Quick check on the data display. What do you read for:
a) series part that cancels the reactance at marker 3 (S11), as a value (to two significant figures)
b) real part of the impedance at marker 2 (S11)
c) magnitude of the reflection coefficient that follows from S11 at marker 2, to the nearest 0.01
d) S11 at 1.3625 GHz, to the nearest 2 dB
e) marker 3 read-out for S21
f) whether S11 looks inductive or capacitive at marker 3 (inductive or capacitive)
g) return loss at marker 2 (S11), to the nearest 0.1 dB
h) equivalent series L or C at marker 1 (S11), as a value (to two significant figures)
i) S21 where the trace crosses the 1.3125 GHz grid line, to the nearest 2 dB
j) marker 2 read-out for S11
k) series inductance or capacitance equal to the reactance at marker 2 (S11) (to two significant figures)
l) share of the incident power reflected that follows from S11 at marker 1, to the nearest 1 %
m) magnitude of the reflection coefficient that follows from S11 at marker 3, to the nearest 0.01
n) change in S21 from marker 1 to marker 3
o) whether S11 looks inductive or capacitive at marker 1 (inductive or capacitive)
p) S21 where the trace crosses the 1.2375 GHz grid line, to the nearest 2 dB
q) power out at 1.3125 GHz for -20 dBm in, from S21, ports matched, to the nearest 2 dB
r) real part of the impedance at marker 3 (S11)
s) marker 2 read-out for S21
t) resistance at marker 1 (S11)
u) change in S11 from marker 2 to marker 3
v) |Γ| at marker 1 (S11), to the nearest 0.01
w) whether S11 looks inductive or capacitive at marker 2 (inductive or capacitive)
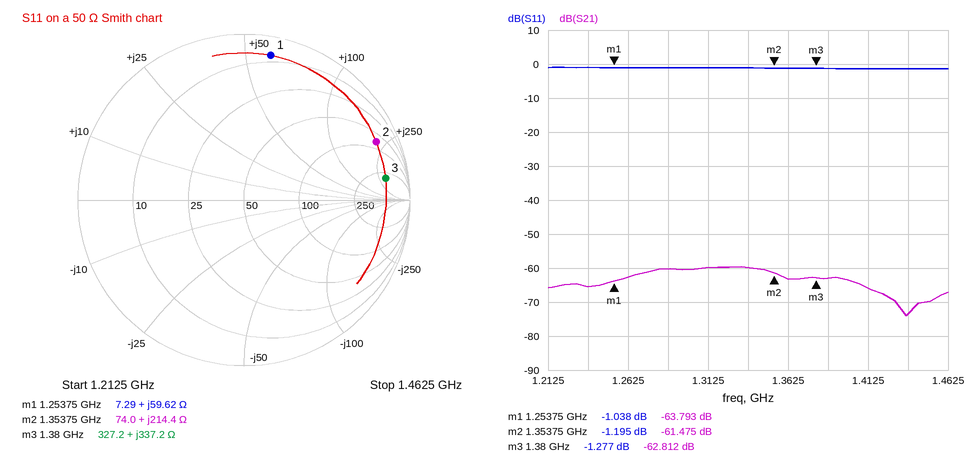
340 fF
74.0 Ω
0.87
-2 dB
-62.812 dB
inductive
1.2 dB
7.6 nH
-60 dB
-1.195 dB
25 nH
79 %
0.86
0.981 dB
inductive
-66 dB
-80 dBm
327.2 Ω
-61.475 dB
7.29 Ω
-0.082 dB
0.89
inductive
